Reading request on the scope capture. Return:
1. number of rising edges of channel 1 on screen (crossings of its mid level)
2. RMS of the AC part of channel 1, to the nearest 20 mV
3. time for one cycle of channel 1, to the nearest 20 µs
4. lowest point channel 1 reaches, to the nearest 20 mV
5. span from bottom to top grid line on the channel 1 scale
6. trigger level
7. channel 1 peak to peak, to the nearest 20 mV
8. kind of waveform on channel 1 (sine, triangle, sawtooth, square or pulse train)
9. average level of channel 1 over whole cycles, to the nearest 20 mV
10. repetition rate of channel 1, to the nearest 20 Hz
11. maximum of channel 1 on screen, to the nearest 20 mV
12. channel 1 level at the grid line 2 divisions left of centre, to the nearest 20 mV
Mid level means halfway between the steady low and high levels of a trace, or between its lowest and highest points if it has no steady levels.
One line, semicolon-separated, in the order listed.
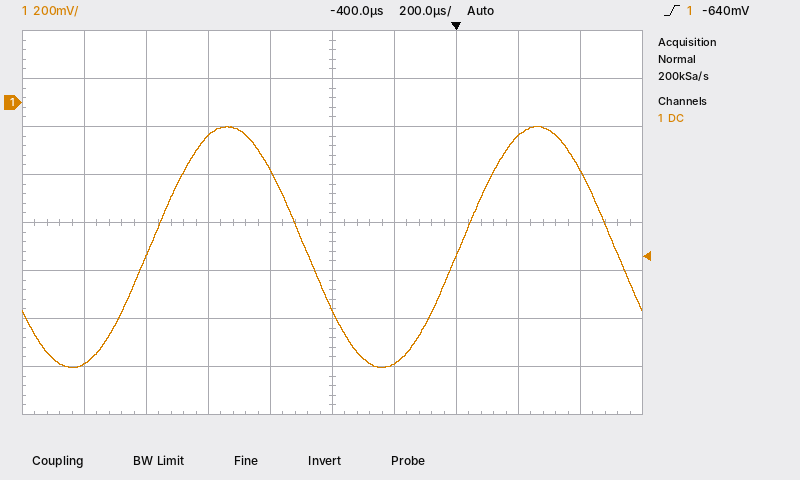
2; 360 mV; 1.00 ms; -1.10 V; 1.6 V; -640 mV; 1.00 V; sine; -600 mV; 1.00 kHz; -100 mV; -140 mV
